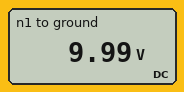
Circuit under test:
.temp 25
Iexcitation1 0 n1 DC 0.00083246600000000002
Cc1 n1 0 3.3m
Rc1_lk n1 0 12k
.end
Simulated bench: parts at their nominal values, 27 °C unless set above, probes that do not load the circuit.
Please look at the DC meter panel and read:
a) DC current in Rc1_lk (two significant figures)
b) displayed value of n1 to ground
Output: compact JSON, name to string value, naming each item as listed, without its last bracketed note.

{"DC current in Rc1_lk": "830 µA", "displayed value of n1 to ground": "9.99 V"}
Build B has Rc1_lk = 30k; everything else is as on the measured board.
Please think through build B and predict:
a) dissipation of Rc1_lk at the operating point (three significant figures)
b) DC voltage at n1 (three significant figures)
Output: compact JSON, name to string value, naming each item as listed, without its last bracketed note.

{"dissipation of Rc1_lk at the operating point": "20.8 mW", "DC voltage at n1": "25.0 V"}
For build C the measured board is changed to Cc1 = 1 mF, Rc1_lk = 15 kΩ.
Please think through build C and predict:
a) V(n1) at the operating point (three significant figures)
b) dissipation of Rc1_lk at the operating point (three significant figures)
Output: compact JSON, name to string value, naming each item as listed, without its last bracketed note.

{"V(n1) at the operating point": "12.5 V", "dissipation of Rc1_lk at the operating point": "10.4 mW"}
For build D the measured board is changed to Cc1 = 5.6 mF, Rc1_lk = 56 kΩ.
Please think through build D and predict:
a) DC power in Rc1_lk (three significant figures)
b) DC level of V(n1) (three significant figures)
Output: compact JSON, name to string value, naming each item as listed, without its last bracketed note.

{"DC power in Rc1_lk": "38.8 mW", "DC level of V(n1)": "46.6 V"}
